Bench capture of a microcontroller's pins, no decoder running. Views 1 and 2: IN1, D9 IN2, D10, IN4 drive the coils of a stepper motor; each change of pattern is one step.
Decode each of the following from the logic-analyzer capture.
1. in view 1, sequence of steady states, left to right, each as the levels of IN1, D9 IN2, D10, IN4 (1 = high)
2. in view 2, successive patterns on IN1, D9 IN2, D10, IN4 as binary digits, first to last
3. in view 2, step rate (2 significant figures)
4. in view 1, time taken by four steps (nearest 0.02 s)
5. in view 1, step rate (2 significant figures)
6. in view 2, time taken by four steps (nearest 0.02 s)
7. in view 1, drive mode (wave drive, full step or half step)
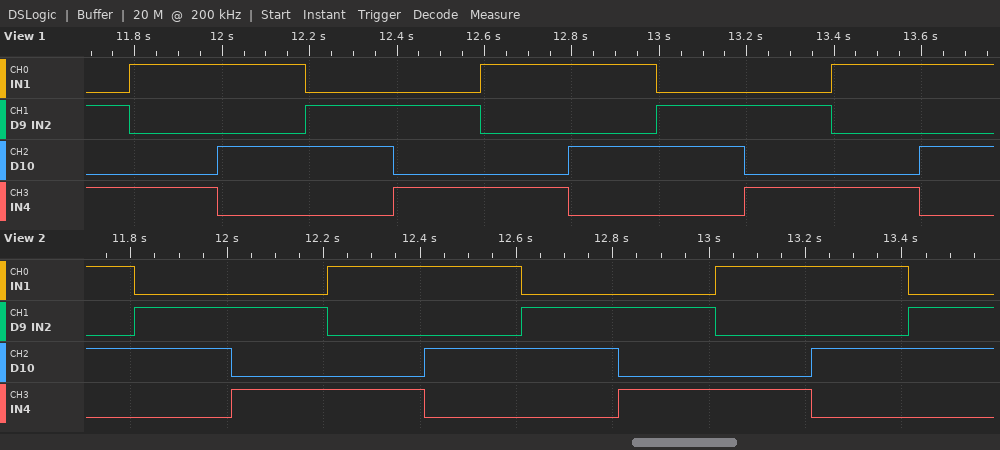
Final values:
0101 1001 1010 0110 0101 1001 1010 0110 0101 1001 1010
1010 0110 0101 1001 1010 0110 0101 1001 1010 0110
5.0 steps/s
0.80 s
5.0 steps/s
0.80 s
full step
